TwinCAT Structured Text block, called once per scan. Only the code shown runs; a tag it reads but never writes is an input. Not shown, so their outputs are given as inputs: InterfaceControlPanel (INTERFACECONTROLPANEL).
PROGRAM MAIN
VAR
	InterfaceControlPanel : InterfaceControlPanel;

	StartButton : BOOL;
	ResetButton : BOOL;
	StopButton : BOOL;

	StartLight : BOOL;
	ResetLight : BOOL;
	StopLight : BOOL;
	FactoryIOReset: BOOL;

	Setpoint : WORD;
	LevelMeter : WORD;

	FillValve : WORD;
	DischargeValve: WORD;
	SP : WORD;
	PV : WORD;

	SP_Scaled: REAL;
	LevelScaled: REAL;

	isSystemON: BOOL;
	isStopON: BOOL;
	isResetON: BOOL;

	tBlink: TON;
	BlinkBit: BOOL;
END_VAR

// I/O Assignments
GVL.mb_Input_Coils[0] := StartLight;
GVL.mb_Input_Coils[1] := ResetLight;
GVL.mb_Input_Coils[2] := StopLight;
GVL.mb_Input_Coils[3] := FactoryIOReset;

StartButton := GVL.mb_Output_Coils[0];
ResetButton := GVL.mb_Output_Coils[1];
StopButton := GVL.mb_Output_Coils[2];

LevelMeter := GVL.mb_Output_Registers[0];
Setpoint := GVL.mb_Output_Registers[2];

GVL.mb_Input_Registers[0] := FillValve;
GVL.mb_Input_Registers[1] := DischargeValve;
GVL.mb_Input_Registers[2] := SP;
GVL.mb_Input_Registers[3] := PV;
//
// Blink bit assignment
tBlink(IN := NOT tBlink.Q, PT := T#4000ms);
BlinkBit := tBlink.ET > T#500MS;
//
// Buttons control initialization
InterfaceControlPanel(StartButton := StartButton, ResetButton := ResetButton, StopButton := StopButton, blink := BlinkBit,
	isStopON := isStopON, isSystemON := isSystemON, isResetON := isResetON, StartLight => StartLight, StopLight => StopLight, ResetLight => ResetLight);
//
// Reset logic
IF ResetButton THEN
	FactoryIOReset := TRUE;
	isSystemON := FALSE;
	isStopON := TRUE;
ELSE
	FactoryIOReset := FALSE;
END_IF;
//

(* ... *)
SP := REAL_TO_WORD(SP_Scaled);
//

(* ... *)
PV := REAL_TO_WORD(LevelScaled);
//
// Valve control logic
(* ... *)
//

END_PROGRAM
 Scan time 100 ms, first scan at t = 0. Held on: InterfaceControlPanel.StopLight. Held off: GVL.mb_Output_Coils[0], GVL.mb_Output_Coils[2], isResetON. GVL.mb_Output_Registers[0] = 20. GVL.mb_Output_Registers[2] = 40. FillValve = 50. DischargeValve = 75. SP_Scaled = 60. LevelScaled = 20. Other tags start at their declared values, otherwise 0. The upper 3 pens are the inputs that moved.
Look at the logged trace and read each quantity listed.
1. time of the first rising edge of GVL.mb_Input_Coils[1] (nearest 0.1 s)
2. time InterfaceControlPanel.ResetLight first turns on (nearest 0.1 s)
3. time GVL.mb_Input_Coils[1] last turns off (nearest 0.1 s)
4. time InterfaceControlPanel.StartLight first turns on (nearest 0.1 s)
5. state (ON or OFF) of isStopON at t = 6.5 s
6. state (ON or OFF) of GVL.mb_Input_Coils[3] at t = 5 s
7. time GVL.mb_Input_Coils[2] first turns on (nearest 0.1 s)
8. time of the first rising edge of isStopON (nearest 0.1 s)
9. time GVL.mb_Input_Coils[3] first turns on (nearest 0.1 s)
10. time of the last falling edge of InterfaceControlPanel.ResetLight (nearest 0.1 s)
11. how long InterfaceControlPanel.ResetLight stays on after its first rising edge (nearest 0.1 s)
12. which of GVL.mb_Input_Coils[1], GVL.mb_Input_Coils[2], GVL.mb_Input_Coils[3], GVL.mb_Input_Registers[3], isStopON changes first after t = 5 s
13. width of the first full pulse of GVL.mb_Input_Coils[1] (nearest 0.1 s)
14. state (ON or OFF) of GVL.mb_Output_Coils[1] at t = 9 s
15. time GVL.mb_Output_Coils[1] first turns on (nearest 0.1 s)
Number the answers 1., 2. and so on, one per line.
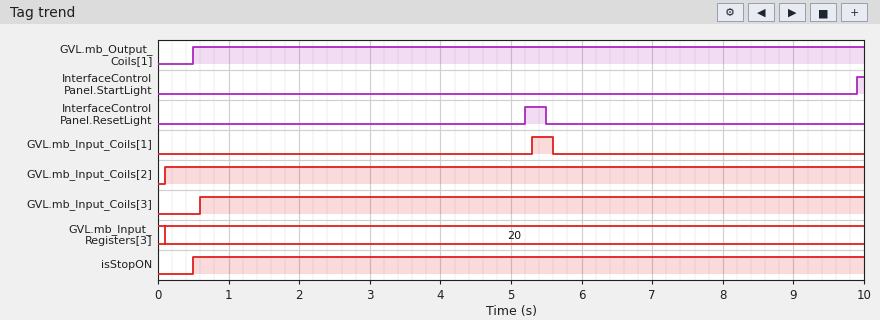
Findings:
1. 5.3 s
2. 5.2 s
3. 5.6 s
4. 9.9 s
5. ON
6. ON
7. 0.1 s
8. 0.5 s
9. 0.6 s
10. 5.5 s
11. 0.3 s
12. GVL.mb_Input_Coils[1]
13. 0.3 s
14. ON
15. 0.5 s
